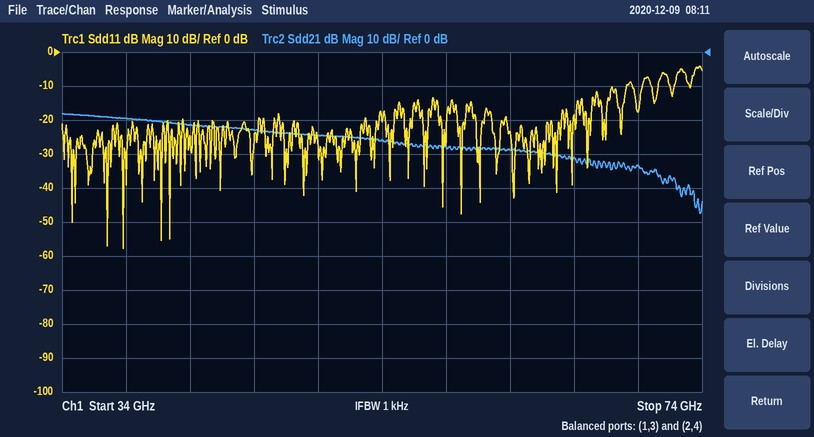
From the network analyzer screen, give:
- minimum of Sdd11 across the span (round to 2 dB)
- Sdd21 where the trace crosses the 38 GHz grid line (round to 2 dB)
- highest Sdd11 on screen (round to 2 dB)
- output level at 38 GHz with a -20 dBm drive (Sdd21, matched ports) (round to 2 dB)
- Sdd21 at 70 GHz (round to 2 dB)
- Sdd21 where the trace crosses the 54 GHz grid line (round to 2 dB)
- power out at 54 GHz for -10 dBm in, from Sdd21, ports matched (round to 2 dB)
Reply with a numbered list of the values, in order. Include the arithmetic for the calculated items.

1. -58 dB
2. -20 dB
3. -4 dB
4. -20 dBm + (-20 dB) = -40 dBm
5. -34 dB
6. -26 dB
7. -10 dBm + (-26 dB) = -36 dBm
